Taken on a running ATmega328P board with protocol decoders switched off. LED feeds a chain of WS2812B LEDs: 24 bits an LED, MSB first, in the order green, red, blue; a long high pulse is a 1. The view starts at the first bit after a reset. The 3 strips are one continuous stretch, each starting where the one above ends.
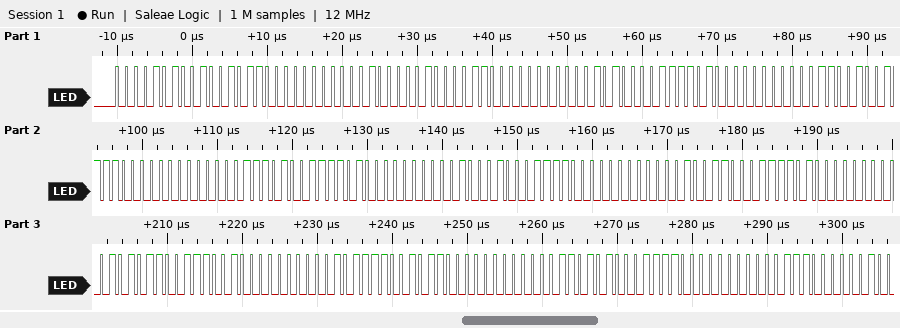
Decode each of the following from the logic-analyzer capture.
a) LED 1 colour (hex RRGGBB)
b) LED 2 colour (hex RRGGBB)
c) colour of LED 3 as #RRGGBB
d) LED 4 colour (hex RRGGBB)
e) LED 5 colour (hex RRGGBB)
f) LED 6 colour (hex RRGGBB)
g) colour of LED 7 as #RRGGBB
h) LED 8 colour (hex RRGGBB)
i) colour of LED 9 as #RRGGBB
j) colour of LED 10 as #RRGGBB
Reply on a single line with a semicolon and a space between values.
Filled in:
#4B0A00; #431000; #3D1400; #3C1900; #3D1D00; #3C2200; #3D2600; #392B00; #2C2F00; #1E3500
